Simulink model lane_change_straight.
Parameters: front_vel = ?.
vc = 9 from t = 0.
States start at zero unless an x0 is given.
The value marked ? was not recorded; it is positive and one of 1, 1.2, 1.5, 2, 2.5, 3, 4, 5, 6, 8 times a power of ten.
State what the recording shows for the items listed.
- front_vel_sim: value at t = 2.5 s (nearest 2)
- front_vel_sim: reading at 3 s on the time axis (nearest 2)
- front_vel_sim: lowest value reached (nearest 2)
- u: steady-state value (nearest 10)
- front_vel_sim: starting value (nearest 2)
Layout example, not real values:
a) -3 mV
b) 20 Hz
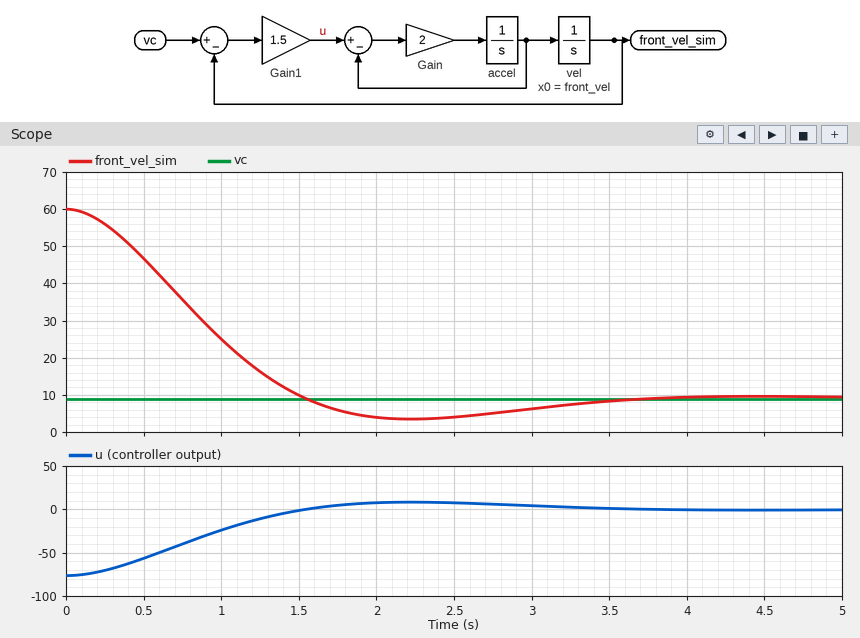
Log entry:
a) 4
b) 6
c) 4
d) 0
e) 60
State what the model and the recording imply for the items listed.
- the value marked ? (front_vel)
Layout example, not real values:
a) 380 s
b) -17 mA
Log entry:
a) 60
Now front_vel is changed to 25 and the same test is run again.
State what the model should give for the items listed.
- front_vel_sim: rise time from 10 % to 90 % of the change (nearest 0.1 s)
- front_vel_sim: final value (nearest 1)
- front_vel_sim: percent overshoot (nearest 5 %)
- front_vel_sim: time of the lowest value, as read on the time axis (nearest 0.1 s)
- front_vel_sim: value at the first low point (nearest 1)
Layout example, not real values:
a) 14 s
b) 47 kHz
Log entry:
a) 1.0 s
b) 9
c) 10 %
d) 2.2 s
e) 7
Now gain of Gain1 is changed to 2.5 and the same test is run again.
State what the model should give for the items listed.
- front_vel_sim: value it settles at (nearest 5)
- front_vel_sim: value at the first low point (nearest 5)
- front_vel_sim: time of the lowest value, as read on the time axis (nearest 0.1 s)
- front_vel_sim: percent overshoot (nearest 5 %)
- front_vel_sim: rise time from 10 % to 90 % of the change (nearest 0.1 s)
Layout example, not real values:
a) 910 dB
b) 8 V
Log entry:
a) 10
b) 0
c) 1.6 s
d) 20 %
e) 0.7 s
